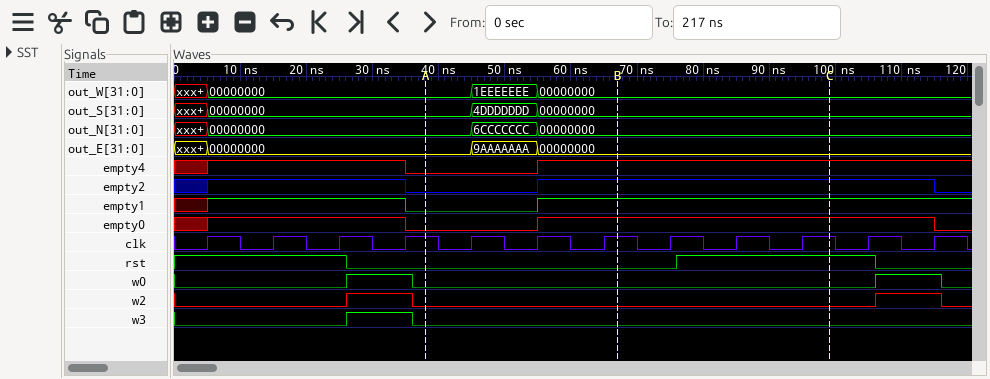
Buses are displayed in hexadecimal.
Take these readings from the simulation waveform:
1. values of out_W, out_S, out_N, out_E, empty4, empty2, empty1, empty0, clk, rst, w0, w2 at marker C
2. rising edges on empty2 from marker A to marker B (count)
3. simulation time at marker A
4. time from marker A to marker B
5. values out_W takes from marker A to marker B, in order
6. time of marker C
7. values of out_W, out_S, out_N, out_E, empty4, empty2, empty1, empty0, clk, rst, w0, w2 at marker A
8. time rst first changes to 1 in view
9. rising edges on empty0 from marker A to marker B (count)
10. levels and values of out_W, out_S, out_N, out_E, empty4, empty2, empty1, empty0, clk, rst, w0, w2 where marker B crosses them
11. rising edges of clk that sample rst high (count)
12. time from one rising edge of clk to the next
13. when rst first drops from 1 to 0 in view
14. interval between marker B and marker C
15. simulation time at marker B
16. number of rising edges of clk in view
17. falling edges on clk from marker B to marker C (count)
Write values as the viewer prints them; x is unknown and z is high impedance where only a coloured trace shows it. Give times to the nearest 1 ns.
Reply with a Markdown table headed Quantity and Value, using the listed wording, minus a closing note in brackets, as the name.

| Quantity | Value |
|---|---|
| values of out_W, out_S, out_N, out_E, empty4, empty2, empty1, empty0, clk, rst, w0, w2 at marker C | out_W=00000000, out_S=00000000, out_N=00000000, out_E=00000000, empty4=1, empty2=1, empty1=1, empty0=1, clk=1, rst=1, w0=0, w2=0 |
| rising edges on empty2 from marker A to marker B | 1 |
| simulation time at marker A | 38 ns |
| time from marker A to marker B | 29 ns |
| values out_W takes from marker A to marker B, in order | 00000000, 1EEEEEEE, 00000000 |
| time of marker C | 99 ns |
| values of out_W, out_S, out_N, out_E, empty4, empty2, empty1, empty0, clk, rst, w0, w2 at marker A | out_W=00000000, out_S=00000000, out_N=00000000, out_E=00000000, empty4=0, empty2=0, empty1=0, empty0=0, clk=1, rst=0, w0=0, w2=0 |
| time rst first changes to 1 in view | 76 ns |
| rising edges on empty0 from marker A to marker B | 1 |
| levels and values of out_W, out_S, out_N, out_E, empty4, empty2, empty1, empty0, clk, rst, w0, w2 where marker B crosses them | out_W=00000000, out_S=00000000, out_N=00000000, out_E=00000000, empty4=1, empty2=1, empty1=1, empty0=1, clk=1, rst=0, w0=0, w2=0 |
| rising edges of clk that sample rst high | 6 |
| time from one rising edge of clk to the next | 10 ns |
| when rst first drops from 1 to 0 in view | 26 ns |
| interval between marker B and marker C | 32 ns |
| simulation time at marker B | 67 ns |
| number of rising edges of clk in view | 12 |
| falling edges on clk from marker B to marker C | 3 |
